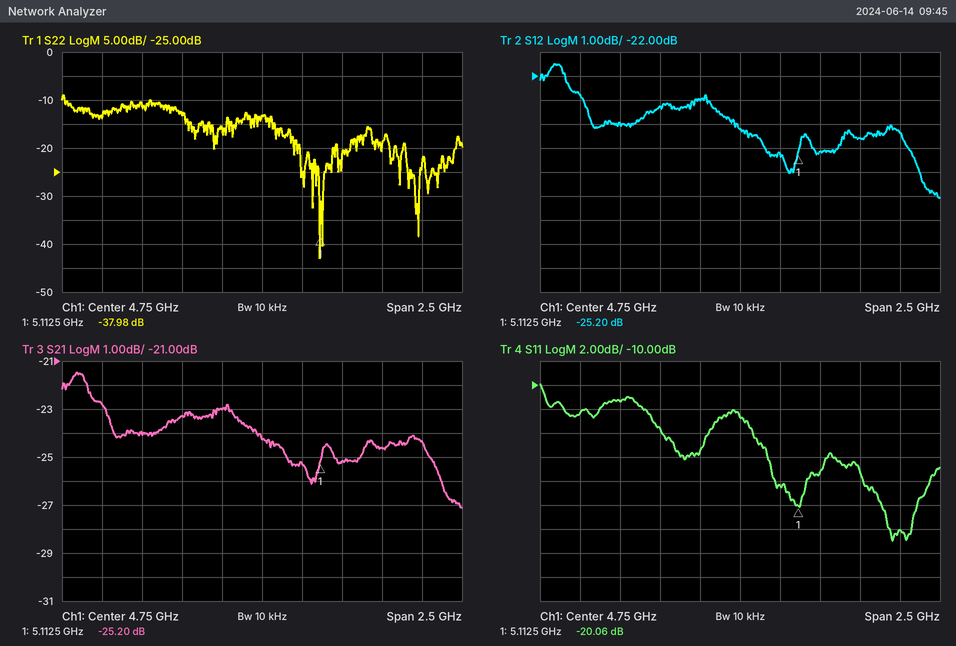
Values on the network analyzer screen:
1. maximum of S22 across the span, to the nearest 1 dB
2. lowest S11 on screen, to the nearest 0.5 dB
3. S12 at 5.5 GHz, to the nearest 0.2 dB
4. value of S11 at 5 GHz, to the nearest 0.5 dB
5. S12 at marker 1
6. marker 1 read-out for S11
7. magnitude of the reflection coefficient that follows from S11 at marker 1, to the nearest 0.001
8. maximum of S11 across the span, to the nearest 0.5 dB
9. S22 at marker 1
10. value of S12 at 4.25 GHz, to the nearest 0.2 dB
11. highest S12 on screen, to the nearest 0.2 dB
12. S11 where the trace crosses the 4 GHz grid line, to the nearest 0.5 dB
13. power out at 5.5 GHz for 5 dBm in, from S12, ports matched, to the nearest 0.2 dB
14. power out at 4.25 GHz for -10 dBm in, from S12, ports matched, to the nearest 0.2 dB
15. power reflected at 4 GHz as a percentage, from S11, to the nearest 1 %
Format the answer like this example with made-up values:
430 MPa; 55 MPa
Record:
-9 dB; -23.0 dB; -24.6 dB; -18.5 dB; -25.20 dB; -20.06 dB; 0.099; -10.0 dB; -37.98 dB; -23.2 dB; -21.4 dB; -11.5 dB; -19.6 dBm; -33.2 dBm; 7 %
